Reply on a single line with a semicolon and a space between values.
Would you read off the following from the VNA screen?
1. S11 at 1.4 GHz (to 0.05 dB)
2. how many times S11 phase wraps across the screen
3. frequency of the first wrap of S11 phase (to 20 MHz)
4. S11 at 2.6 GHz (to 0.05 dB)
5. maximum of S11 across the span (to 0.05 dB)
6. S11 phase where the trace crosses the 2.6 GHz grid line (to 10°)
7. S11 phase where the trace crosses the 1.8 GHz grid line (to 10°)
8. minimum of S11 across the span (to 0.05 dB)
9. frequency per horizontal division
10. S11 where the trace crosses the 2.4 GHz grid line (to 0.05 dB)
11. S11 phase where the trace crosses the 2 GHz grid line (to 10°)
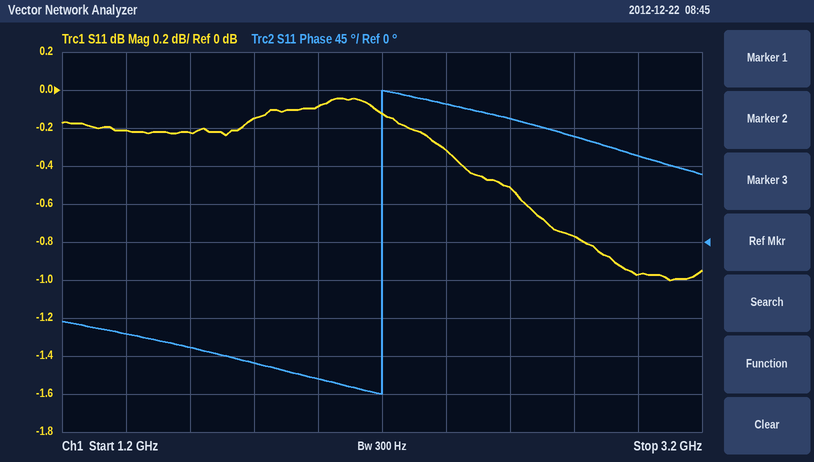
-0.20 dB; 1; 2.20 GHz; -0.50 dB; -0.05 dB; 150°; -140°; -1.00 dB; 200 MHz; -0.30 dB; -160°
